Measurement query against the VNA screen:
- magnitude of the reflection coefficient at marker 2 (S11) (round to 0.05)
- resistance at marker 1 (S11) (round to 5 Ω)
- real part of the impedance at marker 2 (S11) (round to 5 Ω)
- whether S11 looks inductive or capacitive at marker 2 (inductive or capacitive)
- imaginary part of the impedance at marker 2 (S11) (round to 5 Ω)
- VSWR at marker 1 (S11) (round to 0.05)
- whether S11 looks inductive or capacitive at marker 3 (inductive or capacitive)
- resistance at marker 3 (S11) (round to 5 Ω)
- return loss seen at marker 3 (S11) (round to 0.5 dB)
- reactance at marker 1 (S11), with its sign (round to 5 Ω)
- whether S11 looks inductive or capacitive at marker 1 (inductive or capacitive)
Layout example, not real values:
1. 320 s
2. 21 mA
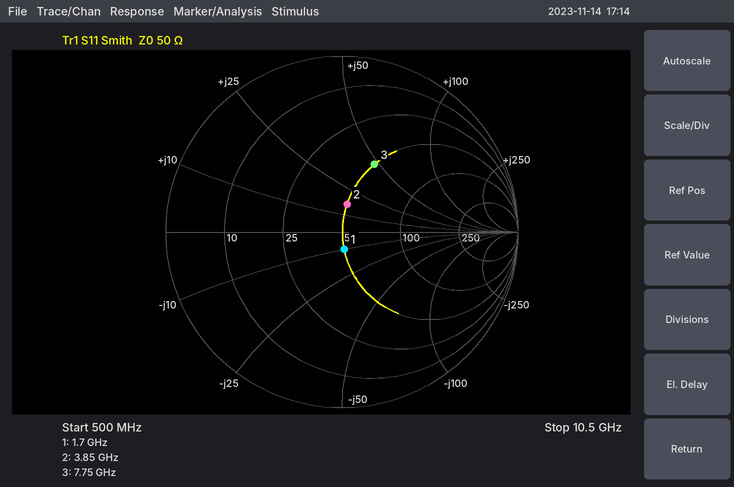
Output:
1. 0.15
2. 50 Ω
3. 50 Ω
4. inductive
5. +15 Ω
6. 1.20
7. inductive
8. 50 Ω
9. 7.5 dB
10. -10 Ω
11. capacitive
